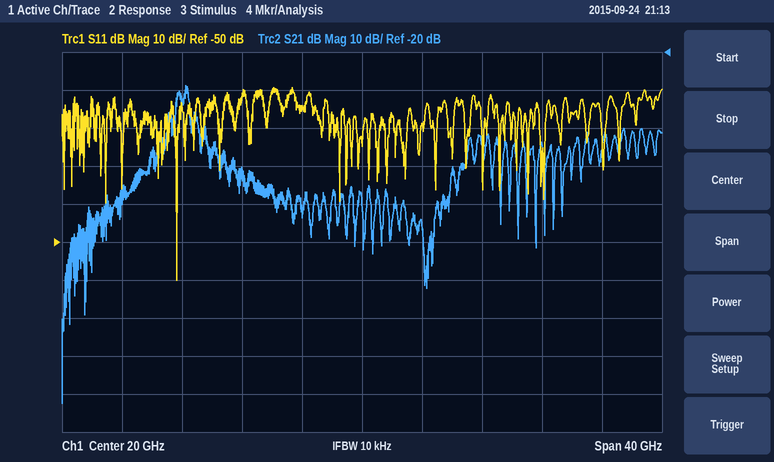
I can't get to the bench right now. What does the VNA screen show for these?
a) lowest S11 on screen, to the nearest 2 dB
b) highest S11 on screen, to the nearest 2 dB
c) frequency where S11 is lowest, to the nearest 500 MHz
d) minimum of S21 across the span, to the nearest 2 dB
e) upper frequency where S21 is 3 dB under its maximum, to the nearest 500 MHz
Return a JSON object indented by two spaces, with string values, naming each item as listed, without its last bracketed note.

{
  "lowest S11 on screen, to the nearest 2 dB": "-60 dB",
  "highest S11 on screen, to the nearest 2 dB": "-10 dB",
  "frequency where S11 is lowest, to the nearest 500 MHz": "7.5 GHz",
  "minimum of S21 across the span, to the nearest 2 dB": "-112 dB",
  "upper frequency where S21 is 3 dB under its maximum, to the nearest 500 MHz": "8.5 GHz"
}
